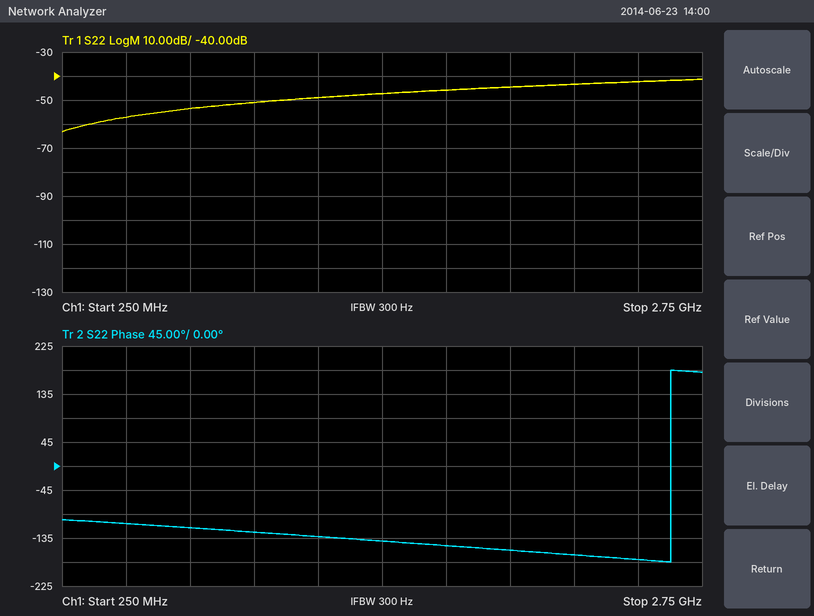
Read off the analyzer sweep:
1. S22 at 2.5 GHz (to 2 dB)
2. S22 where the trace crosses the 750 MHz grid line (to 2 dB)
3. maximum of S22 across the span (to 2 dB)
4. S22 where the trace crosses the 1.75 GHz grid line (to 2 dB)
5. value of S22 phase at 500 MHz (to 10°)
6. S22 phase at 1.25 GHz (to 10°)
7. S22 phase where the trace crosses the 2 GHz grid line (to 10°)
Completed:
-42 dB
-54 dB
-42 dB
-46 dB
-110°
-130°
-160°
